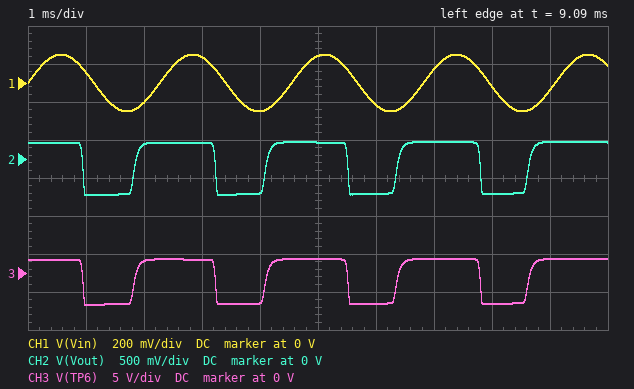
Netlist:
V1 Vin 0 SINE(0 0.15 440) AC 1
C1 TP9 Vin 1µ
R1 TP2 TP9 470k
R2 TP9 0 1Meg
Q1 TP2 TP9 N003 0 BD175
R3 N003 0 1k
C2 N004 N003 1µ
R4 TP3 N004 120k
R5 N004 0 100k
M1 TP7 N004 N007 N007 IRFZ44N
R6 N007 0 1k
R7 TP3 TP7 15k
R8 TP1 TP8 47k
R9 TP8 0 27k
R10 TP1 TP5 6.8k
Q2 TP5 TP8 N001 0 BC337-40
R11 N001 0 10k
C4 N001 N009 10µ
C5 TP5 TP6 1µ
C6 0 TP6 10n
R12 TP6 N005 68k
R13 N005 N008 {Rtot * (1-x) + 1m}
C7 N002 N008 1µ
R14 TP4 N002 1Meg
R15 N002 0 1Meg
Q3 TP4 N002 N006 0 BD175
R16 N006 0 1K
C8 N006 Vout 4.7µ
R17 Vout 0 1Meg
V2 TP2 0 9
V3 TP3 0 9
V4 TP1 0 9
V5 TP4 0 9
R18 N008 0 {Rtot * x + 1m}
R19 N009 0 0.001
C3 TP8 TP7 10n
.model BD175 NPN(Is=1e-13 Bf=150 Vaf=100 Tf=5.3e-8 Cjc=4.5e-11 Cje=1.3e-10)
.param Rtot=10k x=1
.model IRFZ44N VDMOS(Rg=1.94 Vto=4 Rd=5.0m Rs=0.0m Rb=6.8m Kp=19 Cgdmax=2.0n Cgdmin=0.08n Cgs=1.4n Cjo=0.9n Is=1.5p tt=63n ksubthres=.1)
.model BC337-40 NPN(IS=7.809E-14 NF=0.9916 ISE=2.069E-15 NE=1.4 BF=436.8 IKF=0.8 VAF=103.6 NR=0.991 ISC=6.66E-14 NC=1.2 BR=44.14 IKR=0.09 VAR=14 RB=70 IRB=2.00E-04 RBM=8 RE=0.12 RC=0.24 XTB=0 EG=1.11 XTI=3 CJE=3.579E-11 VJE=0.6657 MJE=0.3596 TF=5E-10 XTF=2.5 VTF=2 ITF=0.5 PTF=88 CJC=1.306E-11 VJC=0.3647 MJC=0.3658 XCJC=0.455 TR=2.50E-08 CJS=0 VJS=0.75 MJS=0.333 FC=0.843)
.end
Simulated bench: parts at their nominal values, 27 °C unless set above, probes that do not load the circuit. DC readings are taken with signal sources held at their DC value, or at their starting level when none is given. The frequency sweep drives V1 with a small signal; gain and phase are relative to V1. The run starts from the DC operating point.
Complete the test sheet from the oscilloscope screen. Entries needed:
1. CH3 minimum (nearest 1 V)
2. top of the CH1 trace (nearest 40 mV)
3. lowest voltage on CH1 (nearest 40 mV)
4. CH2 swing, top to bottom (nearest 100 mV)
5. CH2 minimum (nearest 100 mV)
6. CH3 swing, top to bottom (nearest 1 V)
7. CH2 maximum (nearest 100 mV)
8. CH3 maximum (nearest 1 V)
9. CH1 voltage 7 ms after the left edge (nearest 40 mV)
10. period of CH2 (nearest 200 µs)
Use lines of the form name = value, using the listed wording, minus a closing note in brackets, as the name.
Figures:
CH3 minimum = -4 V
top of the CH1 trace = 160 mV
lowest voltage on CH1 = -160 mV
CH2 swing, top to bottom = 700 mV
CH2 minimum = -500 mV
CH3 swing, top to bottom = 6 V
CH2 maximum = 200 mV
CH3 maximum = 2 V
CH1 voltage 7 ms after the left edge = 80 mV
period of CH2 = 2.2 ms
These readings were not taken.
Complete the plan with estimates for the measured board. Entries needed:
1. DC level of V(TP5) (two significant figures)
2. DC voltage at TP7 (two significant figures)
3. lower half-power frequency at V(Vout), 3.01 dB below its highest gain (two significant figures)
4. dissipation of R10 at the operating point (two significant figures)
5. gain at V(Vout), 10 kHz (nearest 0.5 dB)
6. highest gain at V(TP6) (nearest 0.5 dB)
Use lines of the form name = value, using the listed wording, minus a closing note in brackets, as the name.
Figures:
DC level of V(TP5) = 7.2 V
DC voltage at TP7 = 3.5 V
lower half-power frequency at V(Vout), 3.01 dB below its highest gain = 430 Hz
dissipation of R10 at the operating point = 500 µW
gain at V(Vout), 10 kHz = 18.0 dB
highest gain at V(TP6) = 49.0 dB
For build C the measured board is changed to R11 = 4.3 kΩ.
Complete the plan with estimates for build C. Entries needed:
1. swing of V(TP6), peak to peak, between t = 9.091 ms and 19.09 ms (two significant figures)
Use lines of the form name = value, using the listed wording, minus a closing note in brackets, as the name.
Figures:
swing of V(TP6), peak to peak, between t = 9.091 ms and 19.09 ms = 6.2 V
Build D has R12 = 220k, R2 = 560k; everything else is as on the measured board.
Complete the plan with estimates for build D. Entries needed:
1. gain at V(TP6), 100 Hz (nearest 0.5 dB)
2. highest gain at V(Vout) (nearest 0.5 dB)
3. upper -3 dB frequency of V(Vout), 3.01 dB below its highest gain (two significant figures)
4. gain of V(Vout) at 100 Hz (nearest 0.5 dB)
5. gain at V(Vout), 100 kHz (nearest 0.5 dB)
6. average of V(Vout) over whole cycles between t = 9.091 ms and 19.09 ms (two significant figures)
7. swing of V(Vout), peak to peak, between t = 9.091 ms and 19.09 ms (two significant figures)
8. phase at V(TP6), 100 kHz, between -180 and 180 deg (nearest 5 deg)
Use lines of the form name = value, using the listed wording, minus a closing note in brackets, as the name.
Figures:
gain at V(TP6), 100 Hz = 32.0 dB
highest gain at V(Vout) = 21.0 dB
upper -3 dB frequency of V(Vout), 3.01 dB below its highest gain = 3.3 kHz
gain of V(Vout) at 100 Hz = 4.0 dB
gain at V(Vout), 100 kHz = -22.5 dB
average of V(Vout) over whole cycles between t = 9.091 ms and 19.09 ms = -18 mV
swing of V(Vout), peak to peak, between t = 9.091 ms and 19.09 ms = 240 mV
phase at V(TP6), 100 kHz, between -180 and 180 deg = 135 deg
